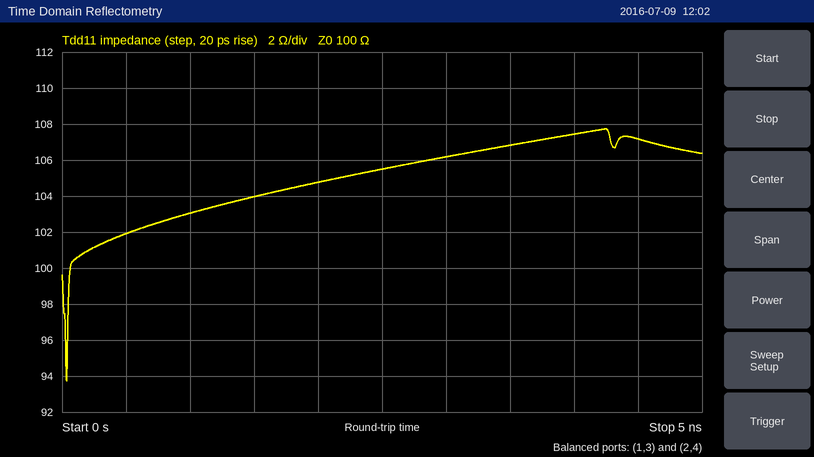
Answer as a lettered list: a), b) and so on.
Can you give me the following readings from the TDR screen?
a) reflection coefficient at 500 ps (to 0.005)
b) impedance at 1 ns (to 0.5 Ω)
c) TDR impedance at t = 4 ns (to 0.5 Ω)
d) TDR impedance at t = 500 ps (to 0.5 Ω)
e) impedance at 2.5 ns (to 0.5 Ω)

a) +0.010
b) 103.0 Ω
c) 107.5 Ω
d) 102.0 Ω
e) 105.5 Ω
